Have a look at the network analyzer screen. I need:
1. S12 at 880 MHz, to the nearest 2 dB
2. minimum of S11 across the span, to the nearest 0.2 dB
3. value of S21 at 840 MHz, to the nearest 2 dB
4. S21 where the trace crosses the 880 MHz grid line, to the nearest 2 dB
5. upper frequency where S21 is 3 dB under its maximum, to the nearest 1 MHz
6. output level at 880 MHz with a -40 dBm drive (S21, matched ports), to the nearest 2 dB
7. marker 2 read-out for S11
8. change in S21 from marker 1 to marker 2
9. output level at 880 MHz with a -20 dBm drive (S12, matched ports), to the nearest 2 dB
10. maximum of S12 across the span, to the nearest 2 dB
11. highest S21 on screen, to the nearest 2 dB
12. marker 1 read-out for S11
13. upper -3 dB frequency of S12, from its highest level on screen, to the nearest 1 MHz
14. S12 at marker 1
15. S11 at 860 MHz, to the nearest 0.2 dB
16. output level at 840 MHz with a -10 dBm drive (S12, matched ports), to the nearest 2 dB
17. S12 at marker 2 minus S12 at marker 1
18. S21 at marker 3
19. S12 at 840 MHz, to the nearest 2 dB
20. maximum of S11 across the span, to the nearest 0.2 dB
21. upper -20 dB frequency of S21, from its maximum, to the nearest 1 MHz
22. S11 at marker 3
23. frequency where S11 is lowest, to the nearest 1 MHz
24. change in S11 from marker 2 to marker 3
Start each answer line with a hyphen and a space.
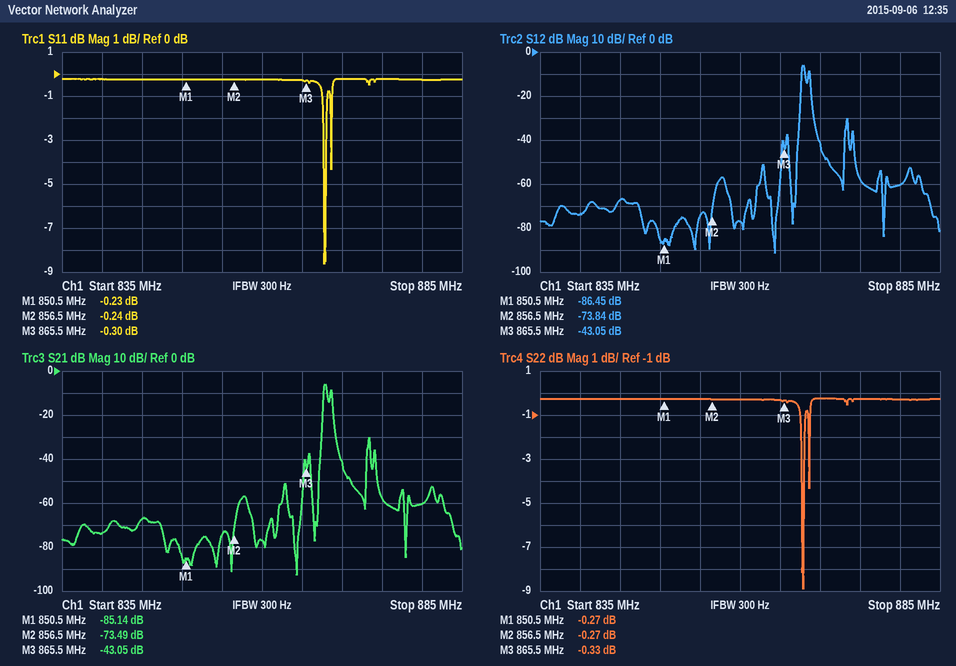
- -60 dB
- -8.6 dB
- -74 dB
- -60 dB
- 868 MHz
- -100 dBm
- -0.24 dB
- 11.65 dB
- -80 dBm
- -6 dB
- -6 dB
- -0.23 dB
- 868 MHz
- -86.45 dB
- -0.2 dB
- -84 dBm
- 12.61 dB
- -43.05 dB
- -74 dB
- -0.2 dB
- 869 MHz
- -0.30 dB
- 868 MHz
- -0.06 dB
